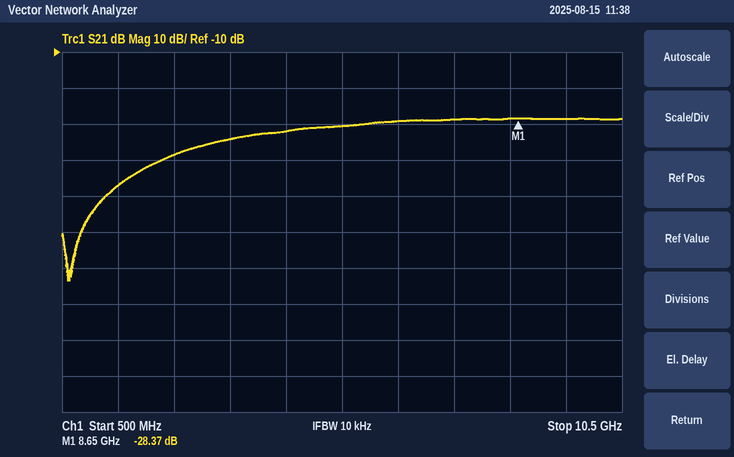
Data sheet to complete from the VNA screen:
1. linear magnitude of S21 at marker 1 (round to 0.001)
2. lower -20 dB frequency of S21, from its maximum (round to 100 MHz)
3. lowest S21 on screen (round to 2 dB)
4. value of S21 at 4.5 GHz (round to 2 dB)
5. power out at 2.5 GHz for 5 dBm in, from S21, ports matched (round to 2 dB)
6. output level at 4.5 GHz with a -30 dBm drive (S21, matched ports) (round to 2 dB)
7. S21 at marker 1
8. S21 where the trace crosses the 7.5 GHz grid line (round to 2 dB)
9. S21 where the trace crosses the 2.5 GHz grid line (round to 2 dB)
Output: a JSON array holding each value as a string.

["0.038", "1.4 GHz", "-74 dB", "-32 dB", "-34 dBm", "-62 dBm", "-28.37 dB", "-28 dB", "-38 dB"]
